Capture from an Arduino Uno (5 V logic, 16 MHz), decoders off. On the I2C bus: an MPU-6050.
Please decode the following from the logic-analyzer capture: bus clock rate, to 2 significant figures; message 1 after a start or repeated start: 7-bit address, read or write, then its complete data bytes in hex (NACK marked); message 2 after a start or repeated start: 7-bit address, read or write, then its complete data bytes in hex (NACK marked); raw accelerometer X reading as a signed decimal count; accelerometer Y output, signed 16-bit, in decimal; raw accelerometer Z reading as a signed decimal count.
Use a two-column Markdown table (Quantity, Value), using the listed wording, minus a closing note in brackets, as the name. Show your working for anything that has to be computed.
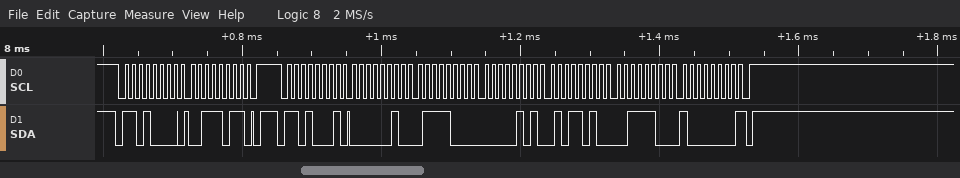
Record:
| Quantity | Value |
|---|---|
| bus clock rate, to 2 significant figures | 100 kHz |
| message 1 after a start or repeated start: 7-bit address, read or write, then its complete data bytes in hex | 0x68 write: 3B |
| message 2 after a start or repeated start: 7-bit address, read or write, then its complete data bytes in hex | 0x68 read: 02 78 05 5A 3C 80 NACK |
| raw accelerometer X reading as a signed decimal count | 0x0278 = 632 |
| accelerometer Y output, signed 16-bit, in decimal | 0x055A = 1370 |
| raw accelerometer Z reading as a signed decimal count | 0x3C80 = 15488 |
